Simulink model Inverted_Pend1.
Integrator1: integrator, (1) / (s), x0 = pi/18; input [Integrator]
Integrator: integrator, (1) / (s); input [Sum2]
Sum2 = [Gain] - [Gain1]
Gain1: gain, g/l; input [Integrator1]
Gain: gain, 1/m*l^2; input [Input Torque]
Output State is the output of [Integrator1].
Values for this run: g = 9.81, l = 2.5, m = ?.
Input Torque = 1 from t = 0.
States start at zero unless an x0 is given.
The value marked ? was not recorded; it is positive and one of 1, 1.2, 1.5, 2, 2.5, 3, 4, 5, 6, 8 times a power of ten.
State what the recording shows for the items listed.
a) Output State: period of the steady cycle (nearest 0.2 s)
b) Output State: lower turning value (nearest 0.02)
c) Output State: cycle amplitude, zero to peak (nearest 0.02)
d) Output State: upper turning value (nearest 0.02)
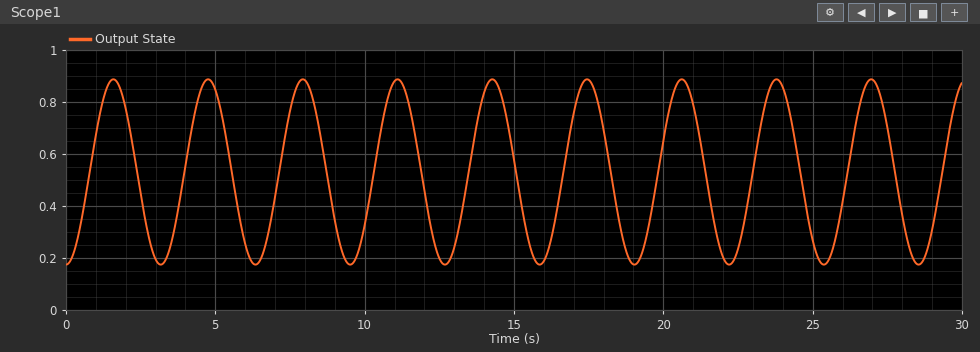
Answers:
3.2 s
0.18
0.36
0.88
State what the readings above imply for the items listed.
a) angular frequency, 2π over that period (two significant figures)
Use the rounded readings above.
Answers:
2.0 rad/s
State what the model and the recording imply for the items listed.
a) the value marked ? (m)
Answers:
3
